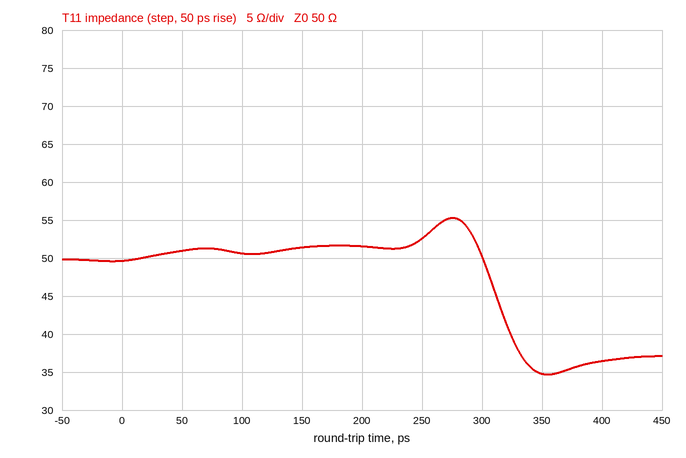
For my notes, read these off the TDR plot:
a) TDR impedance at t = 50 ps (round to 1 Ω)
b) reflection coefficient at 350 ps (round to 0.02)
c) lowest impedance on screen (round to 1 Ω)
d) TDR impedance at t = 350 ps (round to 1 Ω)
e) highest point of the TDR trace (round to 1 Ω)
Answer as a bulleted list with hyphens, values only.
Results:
- 51 Ω
- -0.18
- 35 Ω
- 35 Ω
- 55 Ω
